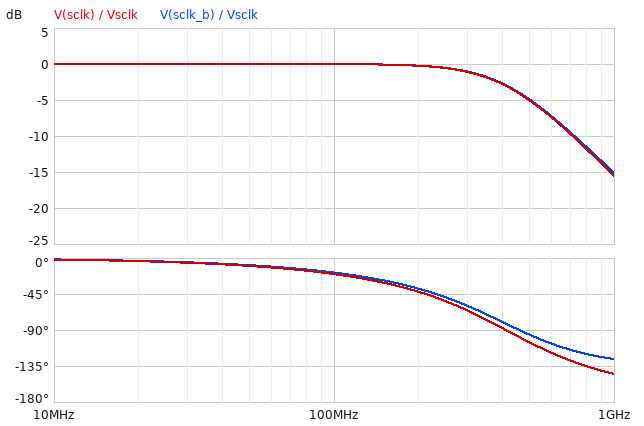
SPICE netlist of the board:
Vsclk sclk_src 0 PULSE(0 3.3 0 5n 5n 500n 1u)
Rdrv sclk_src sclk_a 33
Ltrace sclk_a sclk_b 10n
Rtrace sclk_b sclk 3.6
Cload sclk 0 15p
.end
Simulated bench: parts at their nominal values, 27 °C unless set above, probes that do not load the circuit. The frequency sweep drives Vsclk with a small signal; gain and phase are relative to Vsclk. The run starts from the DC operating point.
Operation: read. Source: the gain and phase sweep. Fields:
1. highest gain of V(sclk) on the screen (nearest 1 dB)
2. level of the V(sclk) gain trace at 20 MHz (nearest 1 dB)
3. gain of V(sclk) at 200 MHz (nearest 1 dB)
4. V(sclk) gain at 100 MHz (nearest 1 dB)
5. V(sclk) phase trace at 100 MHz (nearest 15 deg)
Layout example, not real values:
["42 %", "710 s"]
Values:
["0 dB", "0 dB", "0 dB", "0 dB", "-15 deg"]
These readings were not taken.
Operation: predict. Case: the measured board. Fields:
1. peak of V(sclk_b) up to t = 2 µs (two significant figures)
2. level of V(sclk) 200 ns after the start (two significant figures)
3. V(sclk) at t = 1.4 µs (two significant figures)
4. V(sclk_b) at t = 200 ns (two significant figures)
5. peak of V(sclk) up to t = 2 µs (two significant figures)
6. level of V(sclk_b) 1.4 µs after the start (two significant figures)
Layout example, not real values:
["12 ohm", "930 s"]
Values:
["3.3 V", "3.3 V", "3.3 V", "3.3 V", "3.3 V", "3.3 V"]
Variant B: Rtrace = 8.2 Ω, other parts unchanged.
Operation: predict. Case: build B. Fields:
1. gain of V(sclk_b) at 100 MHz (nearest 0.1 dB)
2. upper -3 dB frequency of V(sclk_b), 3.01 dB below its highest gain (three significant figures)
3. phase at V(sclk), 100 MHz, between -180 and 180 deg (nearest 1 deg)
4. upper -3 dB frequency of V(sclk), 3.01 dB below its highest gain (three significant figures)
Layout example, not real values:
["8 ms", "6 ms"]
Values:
["-0.1 dB", "377 MHz", "-22 deg", "359 MHz"]
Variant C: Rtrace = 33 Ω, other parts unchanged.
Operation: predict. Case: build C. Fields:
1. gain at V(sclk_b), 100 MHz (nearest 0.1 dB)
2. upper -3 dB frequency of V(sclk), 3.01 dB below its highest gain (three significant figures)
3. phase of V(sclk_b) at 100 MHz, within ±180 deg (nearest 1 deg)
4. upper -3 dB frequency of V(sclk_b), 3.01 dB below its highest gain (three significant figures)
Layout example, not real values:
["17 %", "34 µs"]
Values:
["-0.6 dB", "189 MHz", "-16 deg", "305 MHz"]
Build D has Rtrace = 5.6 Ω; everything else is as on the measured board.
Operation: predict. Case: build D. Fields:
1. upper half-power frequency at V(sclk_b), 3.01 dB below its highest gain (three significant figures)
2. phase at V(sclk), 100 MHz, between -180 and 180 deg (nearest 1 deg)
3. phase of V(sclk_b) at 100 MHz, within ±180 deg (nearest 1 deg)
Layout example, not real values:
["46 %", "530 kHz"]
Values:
["397 MHz", "-21 deg", "-18 deg"]
